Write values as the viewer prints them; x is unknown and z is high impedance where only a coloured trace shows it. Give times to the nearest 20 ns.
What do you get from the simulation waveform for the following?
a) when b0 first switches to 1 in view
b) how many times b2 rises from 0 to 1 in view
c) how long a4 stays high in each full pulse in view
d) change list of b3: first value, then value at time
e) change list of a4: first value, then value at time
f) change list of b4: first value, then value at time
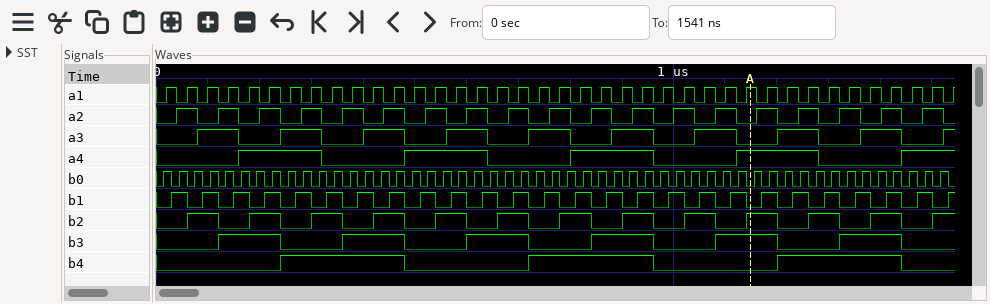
20 ns
13
160 ns, 160 ns, 160 ns, 160 ns
0, 1 at 120 ns, 0 at 240 ns, 1 at 360 ns, 0 at 480 ns, 1 at 600 ns, 0 at 720 ns, 1 at 840 ns, 0 at 960 ns, 1 at 1080 ns, 0 at 1200 ns, 1 at 1320 ns, 0 at 1440 ns
0, 1 at 160 ns, 0 at 320 ns, 1 at 480 ns, 0 at 640 ns, 1 at 800 ns, 0 at 960 ns, 1 at 1120 ns, 0 at 1280 ns, 1 at 1440 ns
0, 1 at 240 ns, 0 at 480 ns, 1 at 720 ns, 0 at 960 ns, 1 at 1200 ns, 0 at 1440 ns
